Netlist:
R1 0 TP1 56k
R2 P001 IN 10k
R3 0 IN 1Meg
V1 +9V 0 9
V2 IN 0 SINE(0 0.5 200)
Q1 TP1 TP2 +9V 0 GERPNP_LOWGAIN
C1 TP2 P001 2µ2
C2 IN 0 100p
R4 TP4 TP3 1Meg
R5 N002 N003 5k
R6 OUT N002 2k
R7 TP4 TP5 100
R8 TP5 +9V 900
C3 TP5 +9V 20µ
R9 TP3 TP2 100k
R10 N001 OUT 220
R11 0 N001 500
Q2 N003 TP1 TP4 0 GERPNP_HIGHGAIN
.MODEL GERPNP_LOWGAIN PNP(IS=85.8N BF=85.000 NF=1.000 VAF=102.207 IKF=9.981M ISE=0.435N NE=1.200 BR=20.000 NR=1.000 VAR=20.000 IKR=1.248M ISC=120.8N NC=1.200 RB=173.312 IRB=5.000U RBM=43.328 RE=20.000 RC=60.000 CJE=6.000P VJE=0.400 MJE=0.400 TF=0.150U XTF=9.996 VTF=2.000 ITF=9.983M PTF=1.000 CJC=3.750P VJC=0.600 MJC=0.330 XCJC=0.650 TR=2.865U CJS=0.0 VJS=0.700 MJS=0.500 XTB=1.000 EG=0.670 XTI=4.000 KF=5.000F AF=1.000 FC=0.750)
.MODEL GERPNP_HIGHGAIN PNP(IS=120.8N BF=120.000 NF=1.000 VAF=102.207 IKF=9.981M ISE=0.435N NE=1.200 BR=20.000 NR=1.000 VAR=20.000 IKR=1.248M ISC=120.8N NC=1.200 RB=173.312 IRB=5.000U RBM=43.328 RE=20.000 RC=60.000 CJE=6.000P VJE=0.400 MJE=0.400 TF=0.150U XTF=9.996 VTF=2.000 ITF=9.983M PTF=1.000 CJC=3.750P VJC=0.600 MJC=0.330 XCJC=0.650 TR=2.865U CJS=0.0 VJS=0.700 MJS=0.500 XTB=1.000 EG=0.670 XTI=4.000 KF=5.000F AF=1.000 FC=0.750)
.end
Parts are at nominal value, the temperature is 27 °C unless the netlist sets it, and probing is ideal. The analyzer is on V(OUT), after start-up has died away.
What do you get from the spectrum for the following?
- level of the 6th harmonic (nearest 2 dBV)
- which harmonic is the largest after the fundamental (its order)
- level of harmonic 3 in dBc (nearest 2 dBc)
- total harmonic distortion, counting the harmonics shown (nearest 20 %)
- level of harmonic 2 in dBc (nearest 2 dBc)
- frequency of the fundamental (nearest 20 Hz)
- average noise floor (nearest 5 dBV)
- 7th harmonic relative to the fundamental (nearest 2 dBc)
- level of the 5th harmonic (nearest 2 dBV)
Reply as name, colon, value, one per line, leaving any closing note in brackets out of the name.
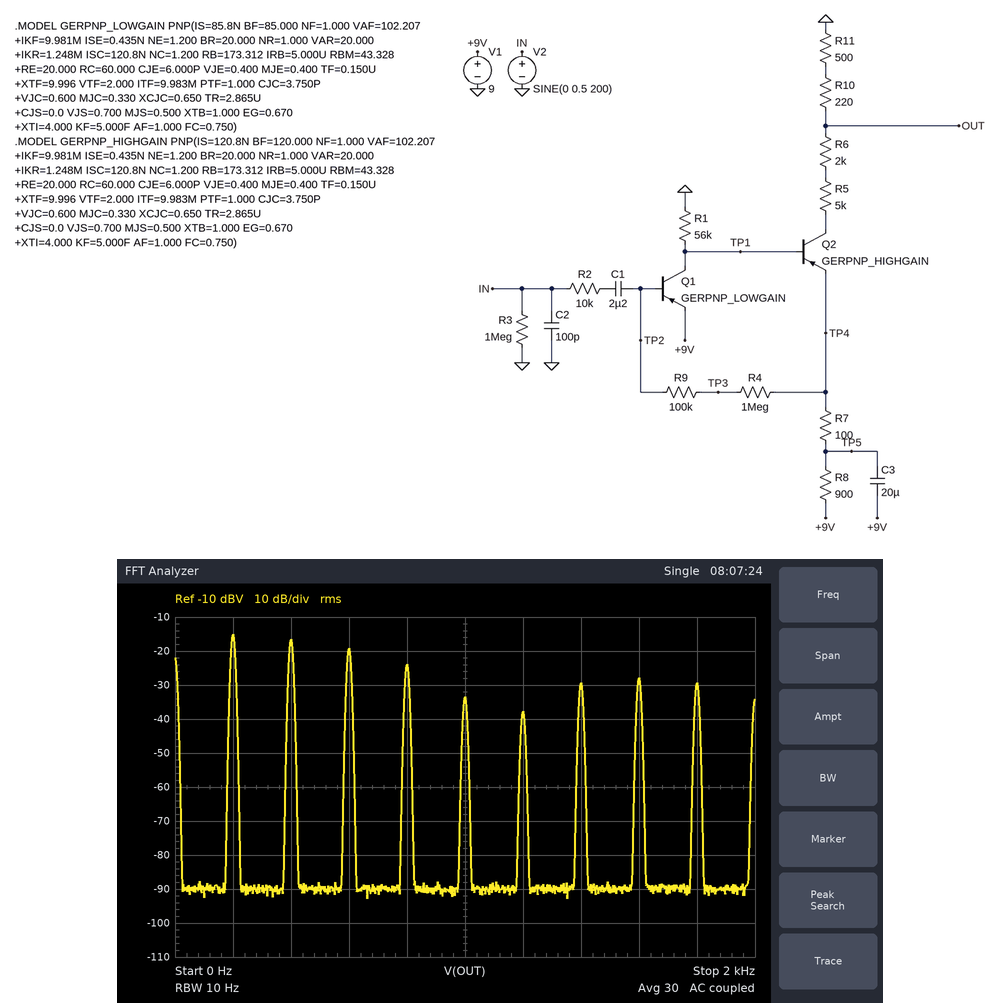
level of the 6th harmonic: -38 dBV
which harmonic is the largest after the fundamental: 2
level of harmonic 3 in dBc: -4 dBc
total harmonic distortion, counting the harmonics shown: 120 %
level of harmonic 2 in dBc: -2 dBc
frequency of the fundamental: 200 Hz
average noise floor: -90 dBV
7th harmonic relative to the fundamental: -14 dBc
level of the 5th harmonic: -34 dBV
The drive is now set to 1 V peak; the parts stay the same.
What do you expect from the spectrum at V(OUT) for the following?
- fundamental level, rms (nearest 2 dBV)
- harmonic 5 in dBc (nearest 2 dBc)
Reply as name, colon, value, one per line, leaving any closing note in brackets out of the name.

fundamental level, rms: -16 dBV
harmonic 5 in dBc: -14 dBc
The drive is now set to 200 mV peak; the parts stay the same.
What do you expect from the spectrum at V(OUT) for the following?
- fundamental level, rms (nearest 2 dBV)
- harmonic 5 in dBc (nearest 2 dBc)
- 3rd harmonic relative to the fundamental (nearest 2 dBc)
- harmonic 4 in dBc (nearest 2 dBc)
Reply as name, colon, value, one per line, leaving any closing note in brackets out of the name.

fundamental level, rms: -14 dBV
harmonic 5 in dBc: -40 dBc
3rd harmonic relative to the fundamental: -6 dBc
harmonic 4 in dBc: -12 dBc
